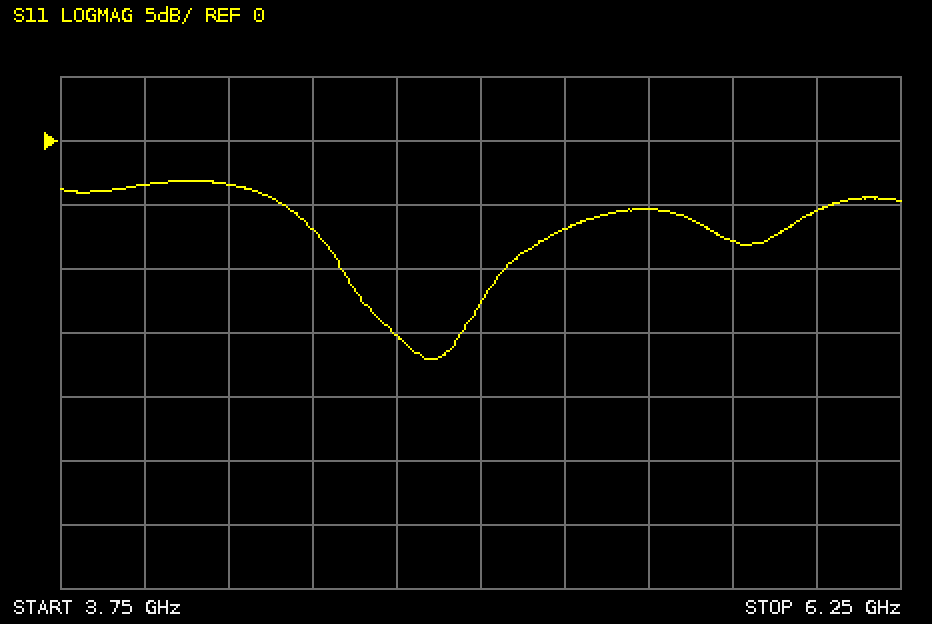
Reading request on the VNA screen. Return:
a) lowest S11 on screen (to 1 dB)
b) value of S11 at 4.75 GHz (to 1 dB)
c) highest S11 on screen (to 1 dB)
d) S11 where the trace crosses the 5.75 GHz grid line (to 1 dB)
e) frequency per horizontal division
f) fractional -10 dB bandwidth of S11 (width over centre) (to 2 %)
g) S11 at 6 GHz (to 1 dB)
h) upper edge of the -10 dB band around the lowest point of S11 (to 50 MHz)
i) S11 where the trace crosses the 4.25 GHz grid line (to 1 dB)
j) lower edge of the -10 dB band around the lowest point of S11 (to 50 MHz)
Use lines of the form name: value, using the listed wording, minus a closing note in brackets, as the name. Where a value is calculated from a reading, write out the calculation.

lowest S11 on screen: -17 dB
value of S11 at 4.75 GHz: -15 dB
highest S11 on screen: -3 dB
S11 where the trace crosses the 5.75 GHz grid line: -8 dB
frequency per horizontal division: 250 MHz
fractional -10 dB bandwidth of S11 (width over centre): 450 MHz / 4.825 GHz ≈ 9.33 %, so 10 % to the nearest 2 %
S11 at 6 GHz: -5 dB
upper edge of the -10 dB band around the lowest point of S11: 5.05 GHz
S11 where the trace crosses the 4.25 GHz grid line: -3 dB
lower edge of the -10 dB band around the lowest point of S11: 4.60 GHz
